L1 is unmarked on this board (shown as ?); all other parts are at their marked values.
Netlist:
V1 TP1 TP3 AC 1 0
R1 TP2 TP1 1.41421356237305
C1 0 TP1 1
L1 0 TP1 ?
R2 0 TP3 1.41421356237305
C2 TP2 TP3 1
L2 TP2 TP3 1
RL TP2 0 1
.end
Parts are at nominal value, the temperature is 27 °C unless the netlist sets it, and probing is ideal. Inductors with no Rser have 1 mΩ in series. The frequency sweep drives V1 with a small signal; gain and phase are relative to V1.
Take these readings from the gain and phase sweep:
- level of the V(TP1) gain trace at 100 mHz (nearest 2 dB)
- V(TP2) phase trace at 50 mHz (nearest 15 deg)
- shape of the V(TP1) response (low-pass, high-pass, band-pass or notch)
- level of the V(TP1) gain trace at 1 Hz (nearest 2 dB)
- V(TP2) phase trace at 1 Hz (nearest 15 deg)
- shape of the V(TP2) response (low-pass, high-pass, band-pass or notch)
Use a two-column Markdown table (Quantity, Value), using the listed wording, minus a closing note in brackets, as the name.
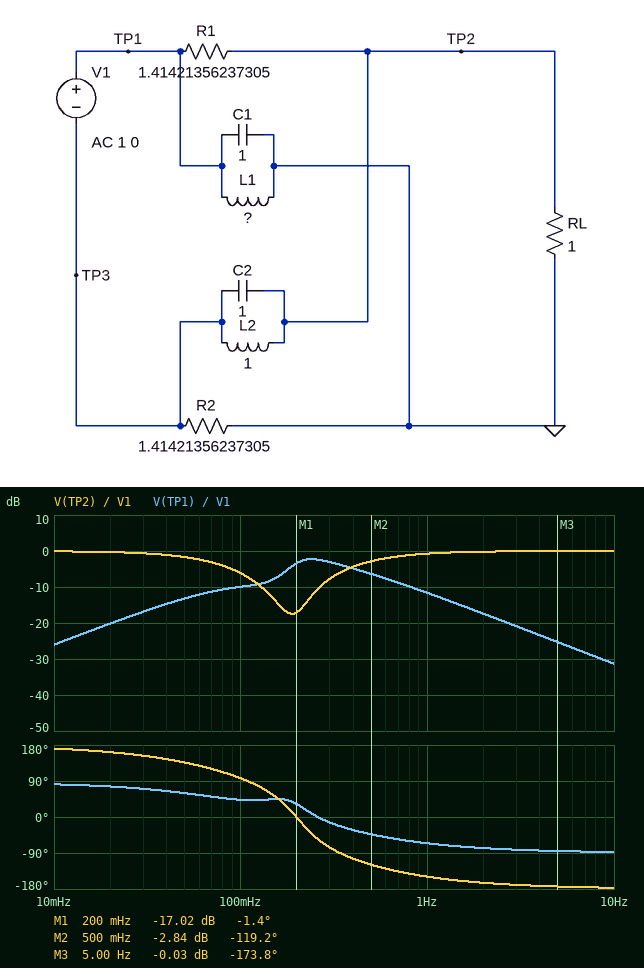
| Quantity | Value |
|---|---|
| level of the V(TP1) gain trace at 100 mHz | -10 dB |
| V(TP2) phase trace at 50 mHz | 135 deg |
| shape of the V(TP1) response | band-pass |
| level of the V(TP1) gain trace at 1 Hz | -12 dB |
| V(TP2) phase trace at 1 Hz | -150 deg |
| shape of the V(TP2) response | notch |
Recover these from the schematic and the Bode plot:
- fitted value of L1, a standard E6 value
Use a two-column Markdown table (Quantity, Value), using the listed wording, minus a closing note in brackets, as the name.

| Quantity | Value |
|---|---|
| fitted value of L1, a standard E6 value | 470 mH |
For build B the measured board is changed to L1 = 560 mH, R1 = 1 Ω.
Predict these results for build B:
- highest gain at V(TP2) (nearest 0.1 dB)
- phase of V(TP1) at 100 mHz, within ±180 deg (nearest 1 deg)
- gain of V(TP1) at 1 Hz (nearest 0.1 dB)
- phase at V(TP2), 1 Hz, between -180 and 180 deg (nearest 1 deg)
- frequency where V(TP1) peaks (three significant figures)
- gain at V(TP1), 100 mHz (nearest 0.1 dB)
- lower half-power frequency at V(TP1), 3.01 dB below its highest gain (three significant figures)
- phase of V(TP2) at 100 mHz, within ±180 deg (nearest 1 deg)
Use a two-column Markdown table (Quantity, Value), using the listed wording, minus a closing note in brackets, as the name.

| Quantity | Value |
|---|---|
| highest gain at V(TP2) | 0 dB |
| phase of V(TP1) at 100 mHz, within ±180 deg | 38 deg |
| gain of V(TP1) at 1 Hz | -11.8 dB |
| phase at V(TP2), 1 Hz, between -180 and 180 deg | -147 deg |
| frequency where V(TP1) peaks | 234 mHz |
| gain at V(TP1), 100 mHz | -9.0 dB |
| lower half-power frequency at V(TP1), 3.01 dB below its highest gain | 156 mHz |
| phase of V(TP2) at 100 mHz, within ±180 deg | 87 deg |
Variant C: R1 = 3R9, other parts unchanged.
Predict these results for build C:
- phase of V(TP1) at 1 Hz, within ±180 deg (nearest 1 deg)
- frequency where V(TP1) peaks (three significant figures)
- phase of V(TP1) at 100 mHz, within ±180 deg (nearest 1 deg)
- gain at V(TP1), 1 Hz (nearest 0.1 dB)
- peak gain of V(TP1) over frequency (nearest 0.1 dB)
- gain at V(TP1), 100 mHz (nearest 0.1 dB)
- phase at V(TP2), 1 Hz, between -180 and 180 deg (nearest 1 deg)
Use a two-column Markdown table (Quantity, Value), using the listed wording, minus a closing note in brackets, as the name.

| Quantity | Value |
|---|---|
| phase of V(TP1) at 1 Hz, within ±180 deg | -68 deg |
| frequency where V(TP1) peaks | 220 mHz |
| phase of V(TP1) at 100 mHz, within ±180 deg | 45 deg |
| gain at V(TP1), 1 Hz | -11.5 dB |
| peak gain of V(TP1) over frequency | -0.7 dB |
| gain at V(TP1), 100 mHz | -9.1 dB |
| phase at V(TP2), 1 Hz, between -180 and 180 deg | -153 deg |
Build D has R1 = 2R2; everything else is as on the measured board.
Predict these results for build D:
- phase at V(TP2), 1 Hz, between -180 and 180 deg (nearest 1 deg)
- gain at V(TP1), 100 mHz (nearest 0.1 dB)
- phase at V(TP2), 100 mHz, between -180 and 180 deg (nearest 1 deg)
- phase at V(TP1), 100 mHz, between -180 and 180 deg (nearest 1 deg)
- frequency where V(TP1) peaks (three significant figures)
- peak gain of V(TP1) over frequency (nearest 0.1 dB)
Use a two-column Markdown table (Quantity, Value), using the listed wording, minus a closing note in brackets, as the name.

| Quantity | Value |
|---|---|
| phase at V(TP2), 1 Hz, between -180 and 180 deg | -151 deg |
| gain at V(TP1), 100 mHz | -9.5 dB |
| phase at V(TP2), 100 mHz, between -180 and 180 deg | 102 deg |
| phase at V(TP1), 100 mHz, between -180 and 180 deg | 44 deg |
| frequency where V(TP1) peaks | 230 mHz |
| peak gain of V(TP1) over frequency | -1.5 dB |
